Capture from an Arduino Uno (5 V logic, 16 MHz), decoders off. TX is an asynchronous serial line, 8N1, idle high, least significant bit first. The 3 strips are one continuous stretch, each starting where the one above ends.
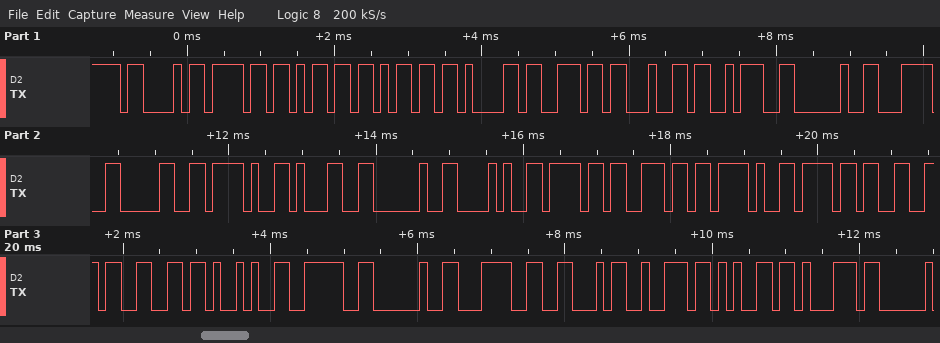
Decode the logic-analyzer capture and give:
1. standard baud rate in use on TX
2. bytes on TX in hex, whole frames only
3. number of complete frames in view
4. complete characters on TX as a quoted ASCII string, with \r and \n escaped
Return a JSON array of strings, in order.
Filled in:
["9600 baud", "43 6F 6D 6D 61 6E 64 3A 20 3C 30 2F 31 20 28 6F 6E 2F 6F 66 66 29 3E 20 3C 46 72 65 71", "29", "\"Command: <0/1 (on/off)> <Freq\""]
